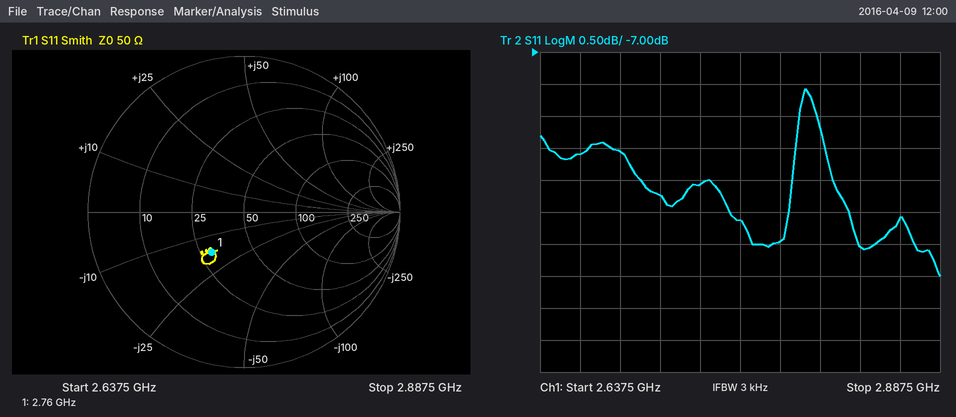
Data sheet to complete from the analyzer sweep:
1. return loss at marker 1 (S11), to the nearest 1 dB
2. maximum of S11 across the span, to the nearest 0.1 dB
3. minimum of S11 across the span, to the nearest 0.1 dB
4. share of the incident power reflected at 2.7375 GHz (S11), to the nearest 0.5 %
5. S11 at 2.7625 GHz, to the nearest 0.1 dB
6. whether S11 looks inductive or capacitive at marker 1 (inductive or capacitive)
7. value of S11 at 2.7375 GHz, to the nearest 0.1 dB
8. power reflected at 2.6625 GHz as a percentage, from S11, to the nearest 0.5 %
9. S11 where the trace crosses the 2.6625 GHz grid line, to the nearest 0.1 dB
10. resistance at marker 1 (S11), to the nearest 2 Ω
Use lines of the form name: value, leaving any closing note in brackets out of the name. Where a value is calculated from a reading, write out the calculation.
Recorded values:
return loss at marker 1 (S11), to the nearest 1 dB: 10 dB
maximum of S11 across the span, to the nearest 0.1 dB: -7.6 dB
minimum of S11 across the span, to the nearest 0.1 dB: -10.5 dB
share of the incident power reflected at 2.7375 GHz (S11), to the nearest 0.5 %: 10^(-9.1/10) ≈ 12.3 %, so 12.5 % to the nearest 0.5 %
S11 at 2.7625 GHz, to the nearest 0.1 dB: -9.6 dB
whether S11 looks inductive or capacitive at marker 1: capacitive
value of S11 at 2.7375 GHz, to the nearest 0.1 dB: -9.1 dB
power reflected at 2.6625 GHz as a percentage, from S11, to the nearest 0.5 %: 10^(-8.6/10) ≈ 13.8 %, so 14.0 % to the nearest 0.5 %
S11 where the trace crosses the 2.6625 GHz grid line, to the nearest 0.1 dB: -8.6 dB
resistance at marker 1 (S11), to the nearest 2 Ω: 30 Ω
